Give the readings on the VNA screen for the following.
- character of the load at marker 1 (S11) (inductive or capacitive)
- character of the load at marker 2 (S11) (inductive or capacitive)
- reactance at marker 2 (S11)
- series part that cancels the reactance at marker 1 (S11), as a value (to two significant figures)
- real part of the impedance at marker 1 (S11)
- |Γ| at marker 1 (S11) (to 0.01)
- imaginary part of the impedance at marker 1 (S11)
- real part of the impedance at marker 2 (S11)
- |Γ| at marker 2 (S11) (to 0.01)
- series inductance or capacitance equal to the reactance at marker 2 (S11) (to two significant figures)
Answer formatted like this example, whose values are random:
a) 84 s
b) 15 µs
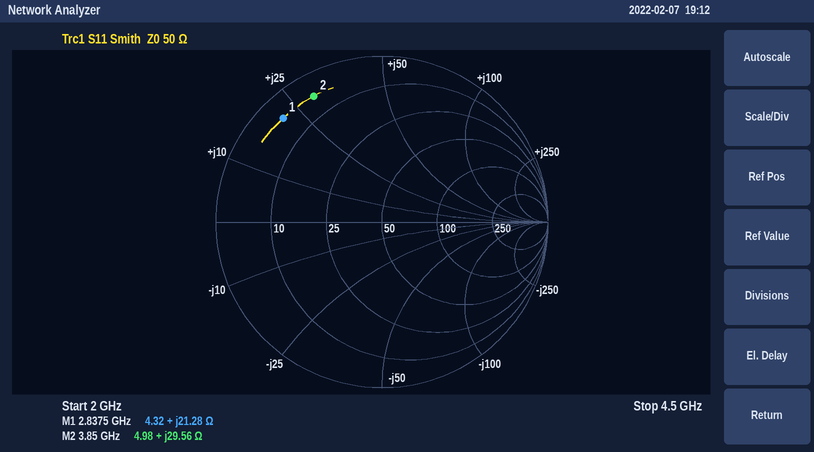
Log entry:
a) inductive
b) inductive
c) +29.56 Ω
d) 2.6 pF
e) 4.32 Ω
f) 0.86
g) +21.28 Ω
h) 4.98 Ω
i) 0.86
j) 1.2 nH
